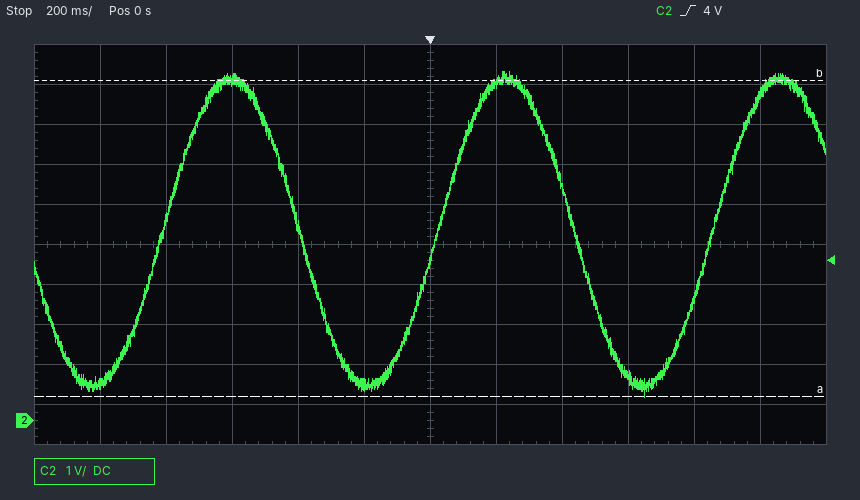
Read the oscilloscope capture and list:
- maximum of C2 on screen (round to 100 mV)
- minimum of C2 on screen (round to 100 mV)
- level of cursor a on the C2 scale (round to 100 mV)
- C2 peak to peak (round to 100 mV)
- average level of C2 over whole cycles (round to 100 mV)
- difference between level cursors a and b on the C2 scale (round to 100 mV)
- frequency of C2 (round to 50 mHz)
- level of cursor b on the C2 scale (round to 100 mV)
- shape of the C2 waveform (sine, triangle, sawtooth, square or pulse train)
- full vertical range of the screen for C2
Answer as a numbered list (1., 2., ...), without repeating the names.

1. 8.7 V
2. 600 mV
3. 600 mV
4. 8.1 V
5. 4.7 V
6. 7.9 V
7. 1.20 Hz
8. 8.5 V
9. sine
10. 10 V
